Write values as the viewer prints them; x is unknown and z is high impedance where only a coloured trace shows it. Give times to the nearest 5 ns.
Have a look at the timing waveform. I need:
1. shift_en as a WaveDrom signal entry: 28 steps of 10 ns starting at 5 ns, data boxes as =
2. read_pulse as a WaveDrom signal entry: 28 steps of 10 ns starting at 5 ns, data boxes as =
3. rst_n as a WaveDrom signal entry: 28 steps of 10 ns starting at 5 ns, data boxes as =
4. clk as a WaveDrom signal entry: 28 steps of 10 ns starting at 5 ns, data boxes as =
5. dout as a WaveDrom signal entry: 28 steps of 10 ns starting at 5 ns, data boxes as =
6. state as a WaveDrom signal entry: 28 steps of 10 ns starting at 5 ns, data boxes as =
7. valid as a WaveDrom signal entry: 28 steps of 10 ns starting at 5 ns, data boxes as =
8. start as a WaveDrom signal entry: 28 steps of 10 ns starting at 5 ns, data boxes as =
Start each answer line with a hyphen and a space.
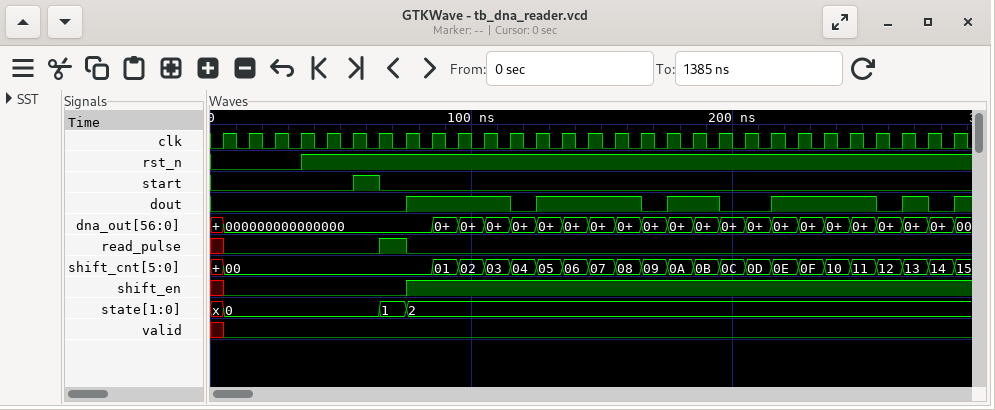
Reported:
- {name: 'shift_en', wave: '0......1....................'}
- {name: 'read_pulse', wave: '0.....10....................'}
- {name: 'rst_n', wave: '0..1........................'}
- {name: 'clk', wave: 'p...........................'}
- {name: 'dout', wave: '0......1...01...01.0.1...010'}
- {name: 'state', wave: '=.....==....................', data: '0 1 2'}
- {name: 'valid', wave: '0...........................'}
- {name: 'start', wave: '0....10.....................'}
